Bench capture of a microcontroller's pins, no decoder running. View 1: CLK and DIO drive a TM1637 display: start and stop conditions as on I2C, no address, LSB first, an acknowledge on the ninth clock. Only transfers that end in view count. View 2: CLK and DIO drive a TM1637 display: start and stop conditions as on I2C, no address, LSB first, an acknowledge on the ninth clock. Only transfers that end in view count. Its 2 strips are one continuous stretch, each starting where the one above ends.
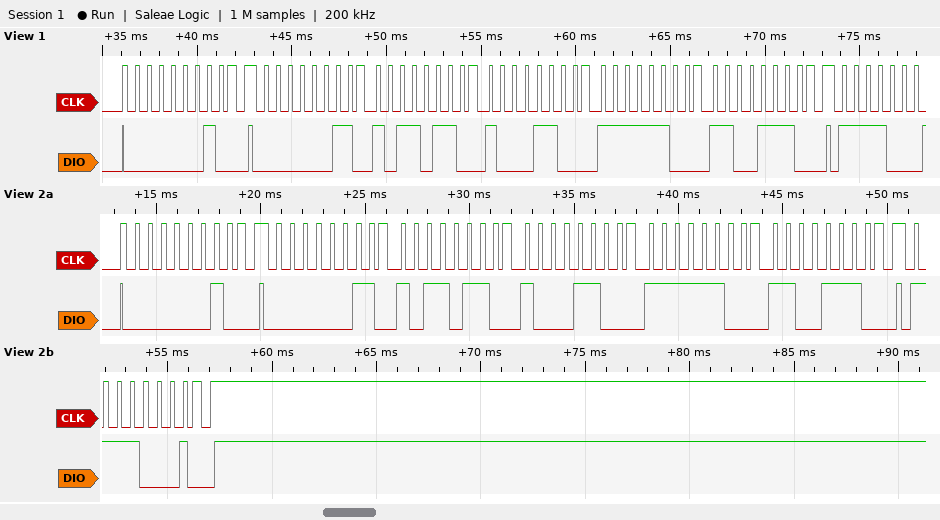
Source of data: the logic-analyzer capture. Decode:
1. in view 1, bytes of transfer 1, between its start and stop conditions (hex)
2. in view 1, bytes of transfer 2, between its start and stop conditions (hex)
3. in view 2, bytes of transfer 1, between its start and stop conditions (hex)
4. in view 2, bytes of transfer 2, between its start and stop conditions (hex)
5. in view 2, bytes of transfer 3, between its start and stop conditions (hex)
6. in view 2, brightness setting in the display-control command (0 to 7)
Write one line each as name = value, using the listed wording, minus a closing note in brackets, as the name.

in view 1, bytes of transfer 1, between its start and stop conditions = 40
in view 1, bytes of transfer 2, between its start and stop conditions = C0 6D 31 3F 73
in view 2, bytes of transfer 1, between its start and stop conditions = 40
in view 2, bytes of transfer 2, between its start and stop conditions = C0 6D 31 3F 73
in view 2, bytes of transfer 3, between its start and stop conditions = 8F
in view 2, brightness setting in the display-control command = 7
